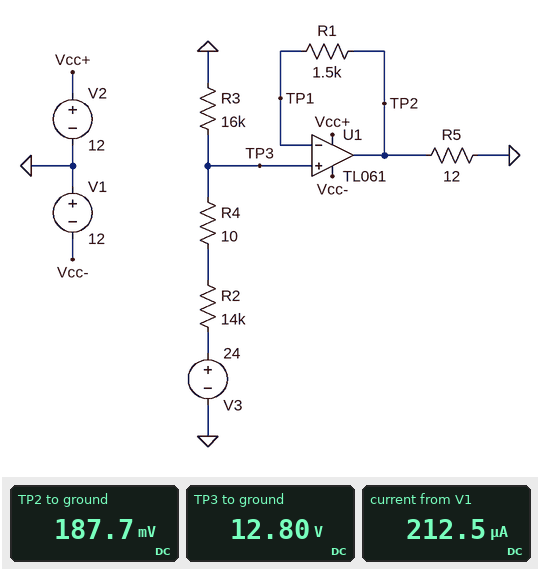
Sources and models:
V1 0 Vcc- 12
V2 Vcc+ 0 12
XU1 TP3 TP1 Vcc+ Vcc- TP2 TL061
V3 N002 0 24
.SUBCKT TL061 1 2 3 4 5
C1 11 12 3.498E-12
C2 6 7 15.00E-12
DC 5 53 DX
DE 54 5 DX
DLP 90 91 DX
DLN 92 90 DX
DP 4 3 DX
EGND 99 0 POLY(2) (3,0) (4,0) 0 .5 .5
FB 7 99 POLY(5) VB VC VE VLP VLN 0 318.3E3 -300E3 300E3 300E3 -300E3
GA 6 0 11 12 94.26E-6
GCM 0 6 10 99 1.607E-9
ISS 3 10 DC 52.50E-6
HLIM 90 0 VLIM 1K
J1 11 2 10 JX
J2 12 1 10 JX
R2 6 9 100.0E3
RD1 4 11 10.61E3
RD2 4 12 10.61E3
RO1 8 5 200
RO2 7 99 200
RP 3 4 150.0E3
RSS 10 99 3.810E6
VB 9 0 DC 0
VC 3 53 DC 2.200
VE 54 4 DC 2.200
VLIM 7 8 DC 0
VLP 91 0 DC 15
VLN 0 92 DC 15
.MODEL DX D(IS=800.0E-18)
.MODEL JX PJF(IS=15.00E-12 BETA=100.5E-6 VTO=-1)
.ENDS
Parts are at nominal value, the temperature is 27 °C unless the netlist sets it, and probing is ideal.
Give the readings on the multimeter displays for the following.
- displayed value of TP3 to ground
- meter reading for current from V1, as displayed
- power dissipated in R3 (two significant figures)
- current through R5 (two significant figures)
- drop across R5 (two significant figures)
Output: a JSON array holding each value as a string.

["12.80 V", "212.5 µA", "10 mW", "16 mA", "190 mV"]
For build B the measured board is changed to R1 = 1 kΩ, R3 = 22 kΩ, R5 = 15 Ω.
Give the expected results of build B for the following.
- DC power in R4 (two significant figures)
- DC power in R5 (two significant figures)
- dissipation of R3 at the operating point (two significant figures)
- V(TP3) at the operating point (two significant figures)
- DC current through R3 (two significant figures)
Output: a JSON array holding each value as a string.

["4.4 µW", "3.7 mW", "9.8 mW", "15 V", "670 µA"]
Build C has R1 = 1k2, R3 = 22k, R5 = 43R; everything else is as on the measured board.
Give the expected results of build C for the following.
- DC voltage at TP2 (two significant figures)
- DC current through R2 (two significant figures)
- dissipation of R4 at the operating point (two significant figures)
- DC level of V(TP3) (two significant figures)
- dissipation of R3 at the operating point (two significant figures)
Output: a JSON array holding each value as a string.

["670 mV", "670 µA", "4.4 µW", "15 V", "9.8 mW"]
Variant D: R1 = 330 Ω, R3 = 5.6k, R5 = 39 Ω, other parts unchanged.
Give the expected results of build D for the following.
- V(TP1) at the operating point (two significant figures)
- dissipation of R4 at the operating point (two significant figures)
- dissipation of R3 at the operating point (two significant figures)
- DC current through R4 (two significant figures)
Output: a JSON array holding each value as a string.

["610 mV", "15 µW", "8.4 mW", "1.2 mA"]
